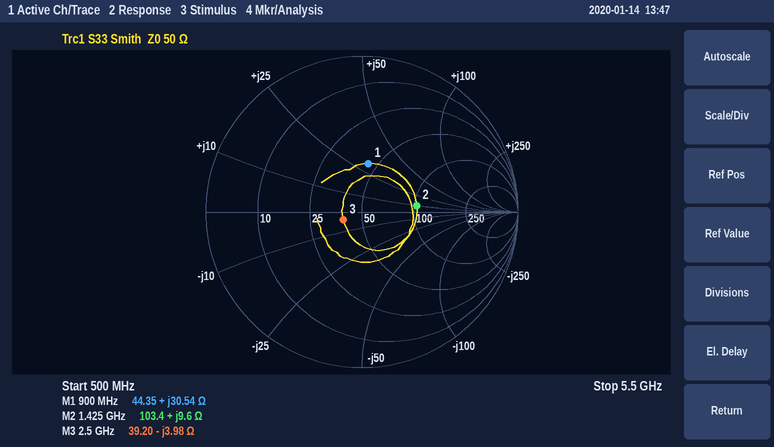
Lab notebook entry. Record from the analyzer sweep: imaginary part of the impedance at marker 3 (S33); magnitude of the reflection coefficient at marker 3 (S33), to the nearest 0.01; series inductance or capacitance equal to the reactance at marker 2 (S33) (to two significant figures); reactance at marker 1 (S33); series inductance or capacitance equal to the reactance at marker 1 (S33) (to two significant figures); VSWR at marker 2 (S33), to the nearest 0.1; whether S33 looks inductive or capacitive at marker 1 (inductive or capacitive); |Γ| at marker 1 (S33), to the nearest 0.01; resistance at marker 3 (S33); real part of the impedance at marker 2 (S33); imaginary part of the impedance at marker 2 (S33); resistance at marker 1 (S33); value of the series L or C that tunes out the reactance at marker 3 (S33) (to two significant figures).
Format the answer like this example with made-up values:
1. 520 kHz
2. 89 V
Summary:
1. -3.98 Ω
2. 0.13
3. 1.1 nH
4. +30.54 Ω
5. 5.4 nH
6. 2.1
7. inductive
8. 0.31
9. 39.20 Ω
10. 103.4 Ω
11. +9.6 Ω
12. 44.35 Ω
13. 250 pH
